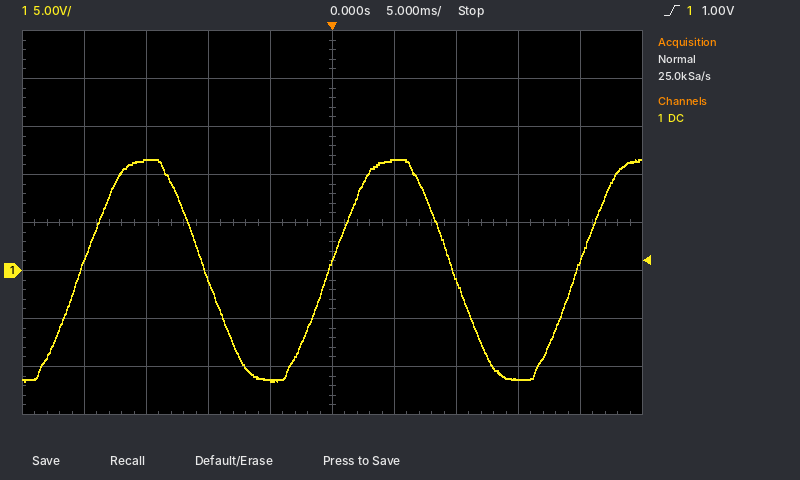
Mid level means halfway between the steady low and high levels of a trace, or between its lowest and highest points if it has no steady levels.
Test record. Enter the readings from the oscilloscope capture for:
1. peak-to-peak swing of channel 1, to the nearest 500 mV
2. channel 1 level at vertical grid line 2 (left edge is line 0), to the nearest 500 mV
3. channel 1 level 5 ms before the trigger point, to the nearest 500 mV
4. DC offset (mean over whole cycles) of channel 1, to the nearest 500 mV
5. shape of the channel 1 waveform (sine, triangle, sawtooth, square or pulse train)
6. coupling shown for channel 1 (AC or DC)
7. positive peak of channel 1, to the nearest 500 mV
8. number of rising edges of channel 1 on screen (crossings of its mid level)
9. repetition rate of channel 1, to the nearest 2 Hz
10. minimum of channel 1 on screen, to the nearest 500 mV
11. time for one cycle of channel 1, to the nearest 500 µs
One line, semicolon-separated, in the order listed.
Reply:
23.0 V; 11.5 V; -11.5 V; 0.0 V; sine; DC; 11.5 V; 3; 50 Hz; -11.5 V; 20.0 ms
